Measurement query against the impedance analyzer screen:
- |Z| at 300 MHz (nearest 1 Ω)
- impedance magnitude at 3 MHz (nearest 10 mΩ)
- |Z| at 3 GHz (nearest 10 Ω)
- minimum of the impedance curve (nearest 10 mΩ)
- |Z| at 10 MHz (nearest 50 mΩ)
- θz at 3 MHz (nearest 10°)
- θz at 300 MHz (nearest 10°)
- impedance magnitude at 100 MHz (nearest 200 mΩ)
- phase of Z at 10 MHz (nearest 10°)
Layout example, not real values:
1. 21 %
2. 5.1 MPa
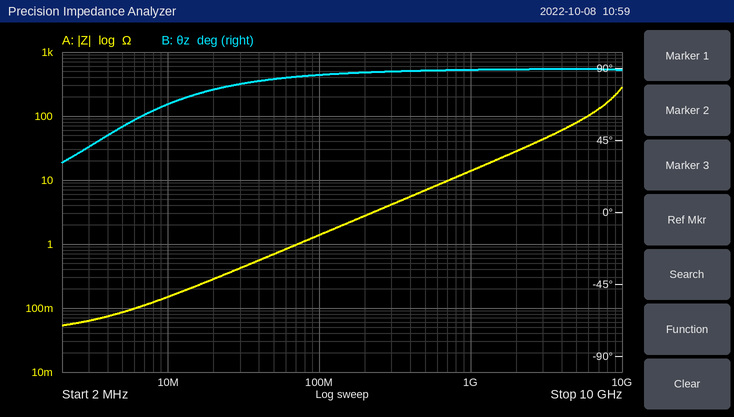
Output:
1. 4 Ω
2. 60 mΩ
3. 40 Ω
4. 50 mΩ
5. 150 mΩ
6. 40°
7. 90°
8. 1.4 Ω
9. 70°
